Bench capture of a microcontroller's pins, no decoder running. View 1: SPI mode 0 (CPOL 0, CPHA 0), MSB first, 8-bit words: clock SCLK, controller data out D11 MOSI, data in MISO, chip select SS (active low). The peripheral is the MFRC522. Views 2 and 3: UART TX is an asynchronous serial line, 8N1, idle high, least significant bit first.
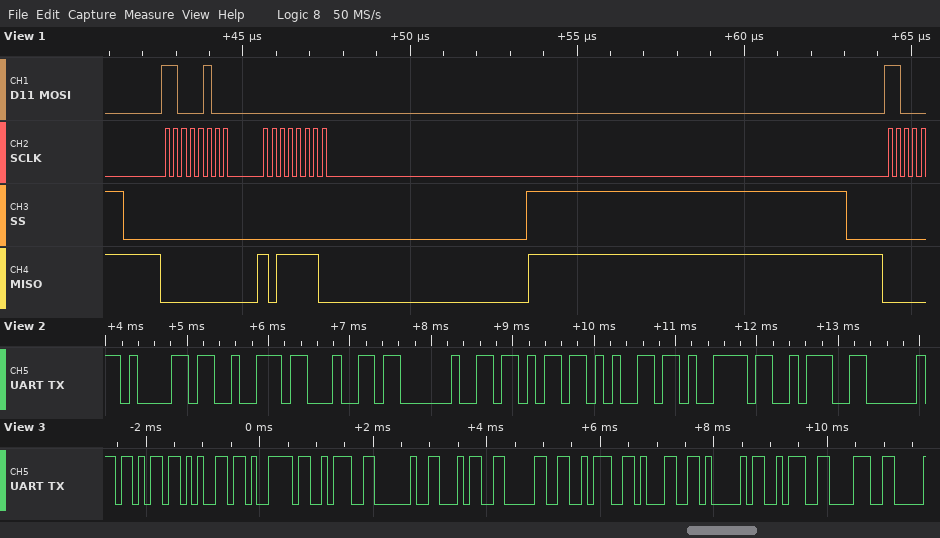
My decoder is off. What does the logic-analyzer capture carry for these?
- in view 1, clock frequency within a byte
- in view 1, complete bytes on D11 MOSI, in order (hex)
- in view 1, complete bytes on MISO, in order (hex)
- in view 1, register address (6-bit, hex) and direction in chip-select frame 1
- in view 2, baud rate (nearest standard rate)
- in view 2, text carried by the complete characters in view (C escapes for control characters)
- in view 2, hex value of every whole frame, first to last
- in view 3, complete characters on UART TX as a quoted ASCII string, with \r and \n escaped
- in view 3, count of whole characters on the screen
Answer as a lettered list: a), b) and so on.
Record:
a) 4 MHz
b) C4 00
c) 00 BE
d) 0x22 read
e) 9600 baud
f) "ard key:"
g) 61 72 64 20 6B 65 79 3A
h) "key: 40:1A:8"
i) 12
